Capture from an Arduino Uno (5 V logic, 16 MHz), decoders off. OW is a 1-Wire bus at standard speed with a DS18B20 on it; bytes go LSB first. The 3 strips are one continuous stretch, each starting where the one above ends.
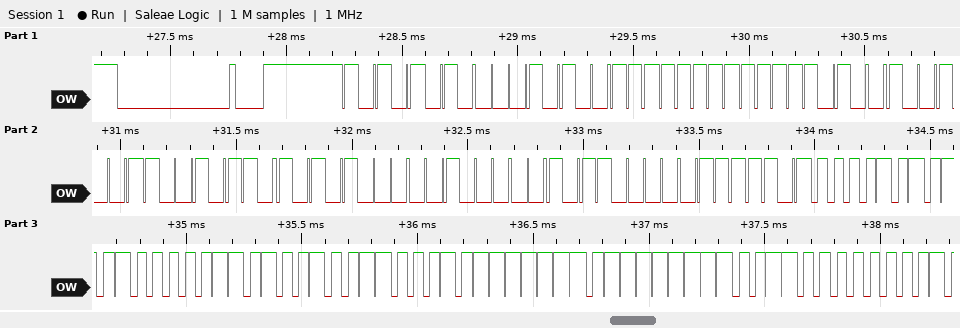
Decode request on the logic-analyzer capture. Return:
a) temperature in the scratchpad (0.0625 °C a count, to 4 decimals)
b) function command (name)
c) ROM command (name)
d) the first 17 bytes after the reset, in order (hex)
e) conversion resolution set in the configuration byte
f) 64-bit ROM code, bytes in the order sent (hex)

85.0000 °C
Read Scratchpad
Match ROM
55 28 FF 5F 92 69 15 04 0D BE 50 05 4B 46 7F FF 0C
12 bits
28 FF 5F 92 69 15 04 0D
